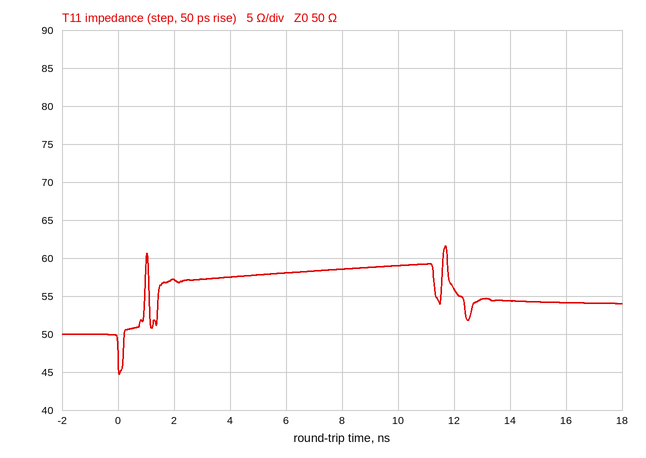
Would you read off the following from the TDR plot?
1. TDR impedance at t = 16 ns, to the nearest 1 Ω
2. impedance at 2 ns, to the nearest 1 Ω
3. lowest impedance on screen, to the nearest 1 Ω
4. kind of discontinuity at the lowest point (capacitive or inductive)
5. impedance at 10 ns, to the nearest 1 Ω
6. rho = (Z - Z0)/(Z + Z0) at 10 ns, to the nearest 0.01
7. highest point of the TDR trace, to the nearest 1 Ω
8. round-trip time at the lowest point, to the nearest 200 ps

54 Ω
57 Ω
45 Ω
capacitive
59 Ω
+0.08
62 Ω
0.0 ns
